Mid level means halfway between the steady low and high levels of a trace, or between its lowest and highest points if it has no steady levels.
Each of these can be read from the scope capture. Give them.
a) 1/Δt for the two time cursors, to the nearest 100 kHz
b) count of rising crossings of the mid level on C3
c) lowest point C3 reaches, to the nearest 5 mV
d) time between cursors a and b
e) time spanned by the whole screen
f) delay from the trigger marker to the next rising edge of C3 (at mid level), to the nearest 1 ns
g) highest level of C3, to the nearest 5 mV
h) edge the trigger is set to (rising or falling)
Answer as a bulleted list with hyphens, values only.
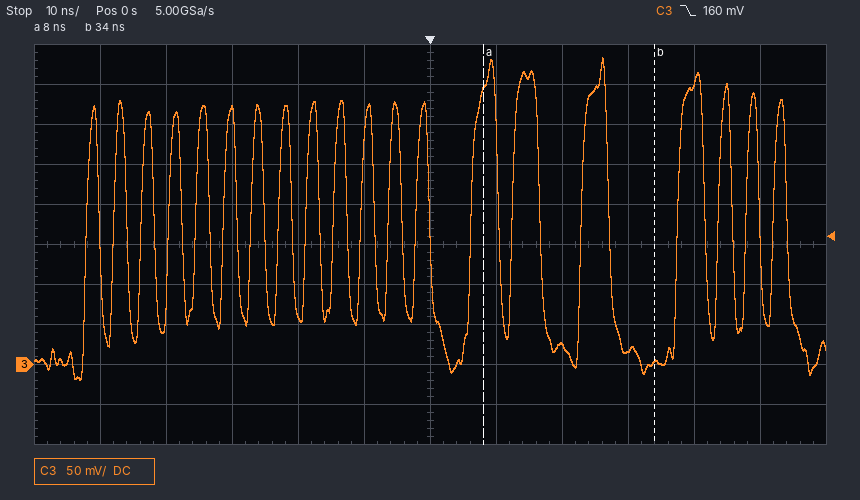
- 38.5 MHz
- 20
- -20 mV
- 26 ns
- 120 ns
- 6 ns
- 385 mV
- falling
